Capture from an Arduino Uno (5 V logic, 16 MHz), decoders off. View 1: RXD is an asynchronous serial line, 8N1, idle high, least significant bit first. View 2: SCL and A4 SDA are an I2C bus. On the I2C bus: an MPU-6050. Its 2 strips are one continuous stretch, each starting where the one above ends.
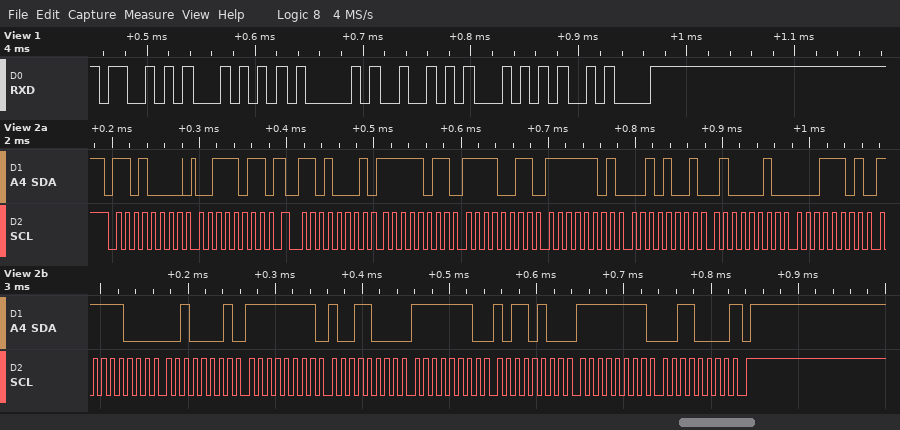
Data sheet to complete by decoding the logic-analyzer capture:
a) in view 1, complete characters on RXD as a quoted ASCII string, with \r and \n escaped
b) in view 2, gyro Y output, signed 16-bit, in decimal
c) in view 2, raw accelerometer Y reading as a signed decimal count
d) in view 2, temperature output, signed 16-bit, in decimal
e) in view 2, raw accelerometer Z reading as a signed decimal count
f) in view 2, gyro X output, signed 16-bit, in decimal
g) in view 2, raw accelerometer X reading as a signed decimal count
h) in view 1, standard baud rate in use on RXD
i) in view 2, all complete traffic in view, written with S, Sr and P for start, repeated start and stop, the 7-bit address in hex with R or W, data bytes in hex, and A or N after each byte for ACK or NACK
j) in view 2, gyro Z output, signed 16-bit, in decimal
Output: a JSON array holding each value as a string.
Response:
["\"START\\n\"", "-332", "-727", "-2015", "16925", "-104", "-1037", "115200 baud", "S 68W A 3B A Sr 68R A FB A F3 A FD A 29 A 42 A 1D A F8 A 21 A FF A 98 A FE A B4 A FF A 30 N P", "-208"]
